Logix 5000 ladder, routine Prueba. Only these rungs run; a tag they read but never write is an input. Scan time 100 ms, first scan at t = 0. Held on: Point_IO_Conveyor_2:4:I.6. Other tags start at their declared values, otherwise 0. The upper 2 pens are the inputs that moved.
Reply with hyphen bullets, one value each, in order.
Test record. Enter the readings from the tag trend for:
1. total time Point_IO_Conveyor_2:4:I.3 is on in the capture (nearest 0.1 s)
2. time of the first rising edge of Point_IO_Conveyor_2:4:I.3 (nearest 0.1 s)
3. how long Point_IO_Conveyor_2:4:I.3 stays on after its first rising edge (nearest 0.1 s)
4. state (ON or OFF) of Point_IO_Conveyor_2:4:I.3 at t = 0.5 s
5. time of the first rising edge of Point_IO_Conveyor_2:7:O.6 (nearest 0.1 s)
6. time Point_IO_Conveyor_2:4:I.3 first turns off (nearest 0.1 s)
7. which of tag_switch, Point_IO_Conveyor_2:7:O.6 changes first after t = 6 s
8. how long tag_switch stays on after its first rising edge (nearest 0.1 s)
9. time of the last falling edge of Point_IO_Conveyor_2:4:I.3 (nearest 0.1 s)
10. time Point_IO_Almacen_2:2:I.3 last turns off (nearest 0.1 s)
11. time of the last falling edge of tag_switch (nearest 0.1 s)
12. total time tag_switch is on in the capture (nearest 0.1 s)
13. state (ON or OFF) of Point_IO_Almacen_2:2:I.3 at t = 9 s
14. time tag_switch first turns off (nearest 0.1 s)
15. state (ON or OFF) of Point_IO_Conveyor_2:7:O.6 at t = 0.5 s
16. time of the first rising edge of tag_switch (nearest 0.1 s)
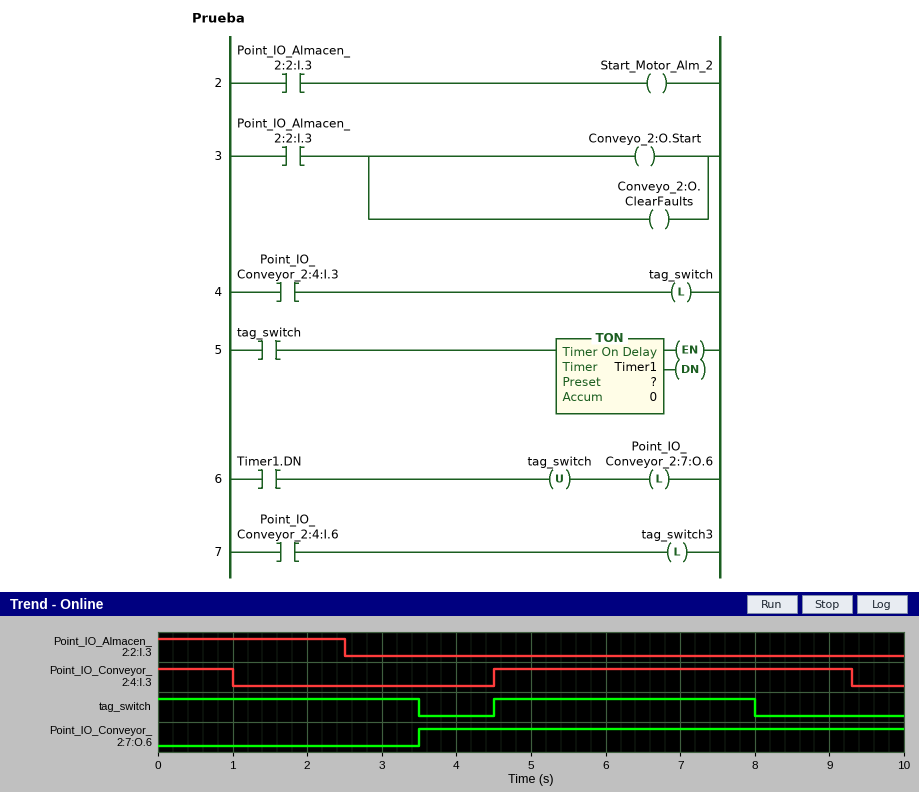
- 5.8 s
- 4.5 s
- 4.8 s
- ON
- 3.5 s
- 1.0 s
- tag_switch
- 3.5 s
- 9.3 s
- 2.5 s
- 8.0 s
- 7.0 s
- OFF
- 3.5 s
- OFF
- 4.5 s
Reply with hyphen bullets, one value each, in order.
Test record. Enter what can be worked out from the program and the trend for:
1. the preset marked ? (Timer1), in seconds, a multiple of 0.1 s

- 3.5 s
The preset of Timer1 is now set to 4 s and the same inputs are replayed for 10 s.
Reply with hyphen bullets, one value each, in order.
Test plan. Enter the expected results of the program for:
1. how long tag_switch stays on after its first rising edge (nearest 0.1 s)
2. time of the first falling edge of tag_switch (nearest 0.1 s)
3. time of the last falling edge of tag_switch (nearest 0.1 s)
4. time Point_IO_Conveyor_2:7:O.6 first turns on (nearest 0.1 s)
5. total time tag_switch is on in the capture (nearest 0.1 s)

- 4.0 s
- 4.0 s
- 8.5 s
- 4.0 s
- 8.0 s
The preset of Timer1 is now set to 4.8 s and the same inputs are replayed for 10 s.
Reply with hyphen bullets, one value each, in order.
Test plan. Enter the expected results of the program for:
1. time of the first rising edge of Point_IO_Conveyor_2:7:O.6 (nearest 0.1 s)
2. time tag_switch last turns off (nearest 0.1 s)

- 4.8 s
- 4.8 s
